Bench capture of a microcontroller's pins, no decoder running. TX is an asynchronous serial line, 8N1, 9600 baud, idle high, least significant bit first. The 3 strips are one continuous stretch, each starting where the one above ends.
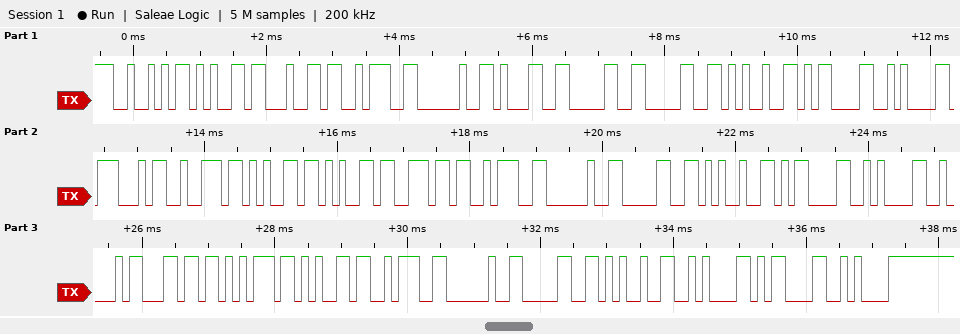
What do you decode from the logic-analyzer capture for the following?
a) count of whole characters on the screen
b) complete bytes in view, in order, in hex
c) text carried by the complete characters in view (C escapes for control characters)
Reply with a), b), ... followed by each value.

a) 33
b) 52 65 64 3A 20 31 30 30 25 0D 0A 47 72 65 65 6E 3A 20 30 25 0D 0A 42 6C 75 65 3A 20 30 25 0A 0D 0A
c) "Red: 100%\r\nGreen: 0%\r\nBlue: 0%\n\r\n"
